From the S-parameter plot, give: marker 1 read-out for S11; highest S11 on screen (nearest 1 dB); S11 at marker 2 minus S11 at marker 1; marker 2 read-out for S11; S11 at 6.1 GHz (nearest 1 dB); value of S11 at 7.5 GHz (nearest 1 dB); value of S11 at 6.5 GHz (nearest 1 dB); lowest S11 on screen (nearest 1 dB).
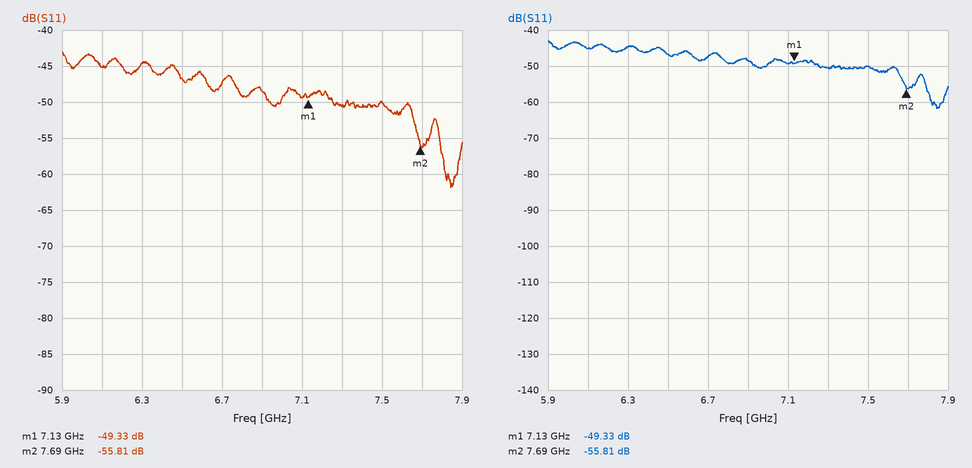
-49.33 dB
-43 dB
-6.48 dB
-55.81 dB
-45 dB
-50 dB
-47 dB
-62 dB
